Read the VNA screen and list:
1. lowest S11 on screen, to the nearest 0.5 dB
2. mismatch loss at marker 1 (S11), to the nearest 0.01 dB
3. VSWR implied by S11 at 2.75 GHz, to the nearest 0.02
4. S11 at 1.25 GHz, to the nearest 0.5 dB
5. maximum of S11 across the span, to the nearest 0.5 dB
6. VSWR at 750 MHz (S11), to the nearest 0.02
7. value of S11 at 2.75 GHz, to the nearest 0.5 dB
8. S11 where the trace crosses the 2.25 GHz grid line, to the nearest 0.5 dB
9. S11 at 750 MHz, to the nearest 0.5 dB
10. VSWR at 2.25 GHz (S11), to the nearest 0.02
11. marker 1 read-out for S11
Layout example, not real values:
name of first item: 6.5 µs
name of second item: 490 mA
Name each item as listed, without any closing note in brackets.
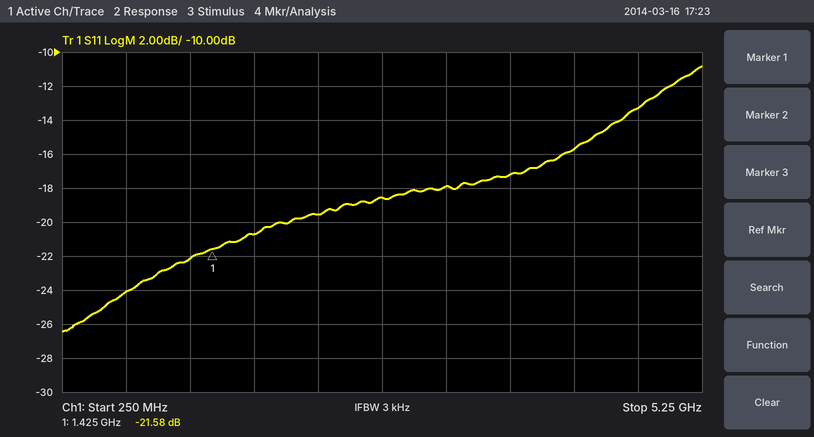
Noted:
lowest S11 on screen, to the nearest 0.5 dB: -26.5 dB
mismatch loss at marker 1 (S11), to the nearest 0.01 dB: 0.03 dB
VSWR implied by S11 at 2.75 GHz, to the nearest 0.02: 1.26
S11 at 1.25 GHz, to the nearest 0.5 dB: -22.0 dB
maximum of S11 across the span, to the nearest 0.5 dB: -11.0 dB
VSWR at 750 MHz (S11), to the nearest 0.02: 1.14
value of S11 at 2.75 GHz, to the nearest 0.5 dB: -18.5 dB
S11 where the trace crosses the 2.25 GHz grid line, to the nearest 0.5 dB: -19.5 dB
S11 at 750 MHz, to the nearest 0.5 dB: -24.0 dB
VSWR at 2.25 GHz (S11), to the nearest 0.02: 1.24
marker 1 read-out for S11: -21.58 dB
